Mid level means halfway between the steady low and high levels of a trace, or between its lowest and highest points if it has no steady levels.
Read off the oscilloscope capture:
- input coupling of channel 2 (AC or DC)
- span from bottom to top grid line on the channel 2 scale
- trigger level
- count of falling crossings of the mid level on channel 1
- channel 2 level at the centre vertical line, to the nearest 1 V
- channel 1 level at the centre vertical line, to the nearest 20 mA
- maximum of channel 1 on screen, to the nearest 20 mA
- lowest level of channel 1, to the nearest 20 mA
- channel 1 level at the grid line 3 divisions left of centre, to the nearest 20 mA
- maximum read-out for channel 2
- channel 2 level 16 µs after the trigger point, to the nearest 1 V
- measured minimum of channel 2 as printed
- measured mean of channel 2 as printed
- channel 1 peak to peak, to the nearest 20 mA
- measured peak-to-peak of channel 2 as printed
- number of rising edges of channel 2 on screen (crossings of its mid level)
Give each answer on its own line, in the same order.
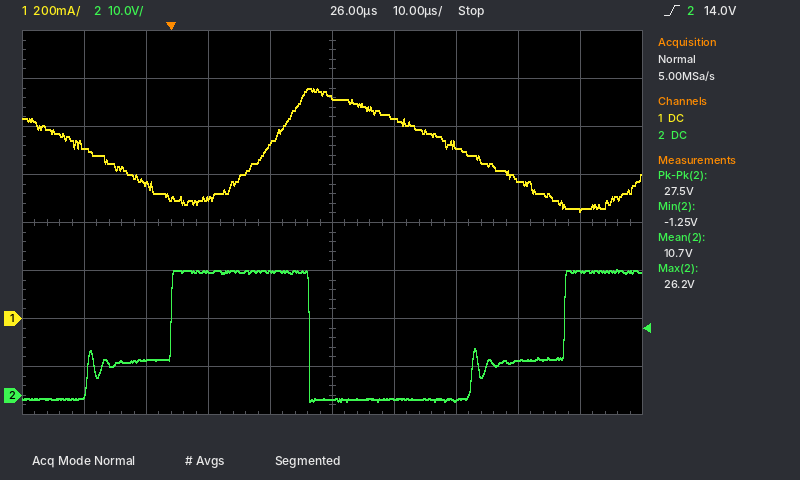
DC
80 V
14.0 V
2
-1 V
920 mA
960 mA
440 mA
560 mA
26.2 V
26 V
-1.25 V
10.7 V
520 mA
27.5 V
2
